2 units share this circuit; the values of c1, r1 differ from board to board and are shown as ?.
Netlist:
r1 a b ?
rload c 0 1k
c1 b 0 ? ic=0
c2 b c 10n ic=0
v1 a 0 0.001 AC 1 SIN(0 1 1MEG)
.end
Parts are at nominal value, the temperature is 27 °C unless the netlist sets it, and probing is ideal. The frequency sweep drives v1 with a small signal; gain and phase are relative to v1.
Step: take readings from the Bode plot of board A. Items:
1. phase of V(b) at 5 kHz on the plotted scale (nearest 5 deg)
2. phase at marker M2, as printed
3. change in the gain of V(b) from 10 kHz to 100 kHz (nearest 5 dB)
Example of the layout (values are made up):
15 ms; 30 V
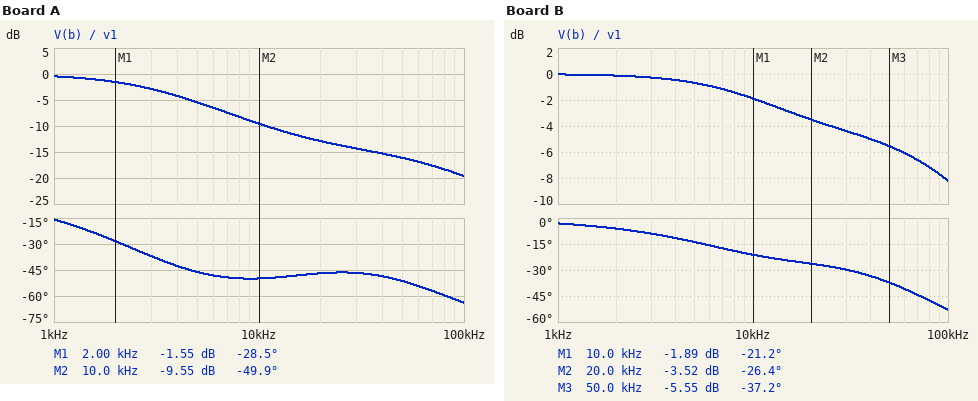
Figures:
-45 deg; -49.9 deg; -10 dB
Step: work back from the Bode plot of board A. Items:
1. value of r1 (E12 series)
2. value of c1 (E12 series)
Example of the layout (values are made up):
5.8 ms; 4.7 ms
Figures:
3.3 kΩ; 3.9 nF
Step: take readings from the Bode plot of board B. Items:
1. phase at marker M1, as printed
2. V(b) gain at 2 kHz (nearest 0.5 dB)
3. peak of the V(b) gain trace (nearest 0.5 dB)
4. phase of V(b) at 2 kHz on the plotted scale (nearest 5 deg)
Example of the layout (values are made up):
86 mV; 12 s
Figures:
-21.2 deg; 0 dB; 0 dB; -5 deg
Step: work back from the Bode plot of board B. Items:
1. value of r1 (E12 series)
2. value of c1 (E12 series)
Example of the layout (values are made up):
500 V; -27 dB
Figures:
560 Ω; 5.6 nF
